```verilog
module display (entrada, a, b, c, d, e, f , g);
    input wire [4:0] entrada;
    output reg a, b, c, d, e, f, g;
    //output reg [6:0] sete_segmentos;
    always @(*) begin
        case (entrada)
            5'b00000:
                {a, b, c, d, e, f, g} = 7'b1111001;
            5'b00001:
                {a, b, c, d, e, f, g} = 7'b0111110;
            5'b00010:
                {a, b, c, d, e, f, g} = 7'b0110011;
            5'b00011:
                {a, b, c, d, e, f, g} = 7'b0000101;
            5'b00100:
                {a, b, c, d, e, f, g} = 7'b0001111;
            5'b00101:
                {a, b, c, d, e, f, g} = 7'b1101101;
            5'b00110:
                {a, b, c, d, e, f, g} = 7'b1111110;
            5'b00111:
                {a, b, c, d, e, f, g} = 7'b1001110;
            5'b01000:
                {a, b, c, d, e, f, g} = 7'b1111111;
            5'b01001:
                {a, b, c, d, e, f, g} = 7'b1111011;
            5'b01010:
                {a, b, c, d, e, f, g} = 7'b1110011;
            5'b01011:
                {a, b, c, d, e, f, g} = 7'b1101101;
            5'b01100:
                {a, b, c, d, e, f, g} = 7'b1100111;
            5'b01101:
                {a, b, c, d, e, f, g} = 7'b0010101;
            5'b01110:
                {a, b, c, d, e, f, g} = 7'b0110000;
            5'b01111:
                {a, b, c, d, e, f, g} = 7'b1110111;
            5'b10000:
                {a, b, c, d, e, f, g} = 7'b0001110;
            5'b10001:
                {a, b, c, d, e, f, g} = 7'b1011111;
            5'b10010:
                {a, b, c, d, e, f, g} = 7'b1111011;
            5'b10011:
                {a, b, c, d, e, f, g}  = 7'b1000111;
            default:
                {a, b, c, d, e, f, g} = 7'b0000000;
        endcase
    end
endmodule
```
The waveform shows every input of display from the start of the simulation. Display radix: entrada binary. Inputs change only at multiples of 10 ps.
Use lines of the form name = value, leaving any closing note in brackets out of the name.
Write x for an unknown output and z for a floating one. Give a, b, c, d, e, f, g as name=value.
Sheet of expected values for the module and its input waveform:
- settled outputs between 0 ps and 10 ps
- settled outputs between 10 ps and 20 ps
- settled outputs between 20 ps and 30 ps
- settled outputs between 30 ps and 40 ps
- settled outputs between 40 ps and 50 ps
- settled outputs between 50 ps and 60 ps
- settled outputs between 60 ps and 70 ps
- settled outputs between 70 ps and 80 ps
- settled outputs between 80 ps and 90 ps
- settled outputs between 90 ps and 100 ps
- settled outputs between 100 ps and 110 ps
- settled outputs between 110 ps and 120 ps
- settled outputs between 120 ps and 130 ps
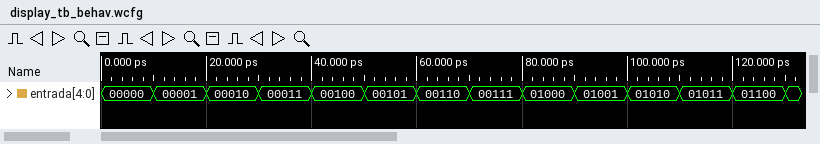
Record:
settled outputs between 0 ps and 10 ps = a=1, b=1, c=1, d=1, e=0, f=0, g=1
settled outputs between 10 ps and 20 ps = a=0, b=1, c=1, d=1, e=1, f=1, g=0
settled outputs between 20 ps and 30 ps = a=0, b=1, c=1, d=0, e=0, f=1, g=1
settled outputs between 30 ps and 40 ps = a=0, b=0, c=0, d=0, e=1, f=0, g=1
settled outputs between 40 ps and 50 ps = a=0, b=0, c=0, d=1, e=1, f=1, g=1
settled outputs between 50 ps and 60 ps = a=1, b=1, c=0, d=1, e=1, f=0, g=1
settled outputs between 60 ps and 70 ps = a=1, b=1, c=1, d=1, e=1, f=1, g=0
settled outputs between 70 ps and 80 ps = a=1, b=0, c=0, d=1, e=1, f=1, g=0
settled outputs between 80 ps and 90 ps = a=1, b=1, c=1, d=1, e=1, f=1, g=1
settled outputs between 90 ps and 100 ps = a=1, b=1, c=1, d=1, e=0, f=1, g=1
settled outputs between 100 ps and 110 ps = a=1, b=1, c=1, d=0, e=0, f=1, g=1
settled outputs between 110 ps and 120 ps = a=1, b=1, c=0, d=1, e=1, f=0, g=1
settled outputs between 120 ps and 130 ps = a=1, b=1, c=0, d=0, e=1, f=1, g=1
